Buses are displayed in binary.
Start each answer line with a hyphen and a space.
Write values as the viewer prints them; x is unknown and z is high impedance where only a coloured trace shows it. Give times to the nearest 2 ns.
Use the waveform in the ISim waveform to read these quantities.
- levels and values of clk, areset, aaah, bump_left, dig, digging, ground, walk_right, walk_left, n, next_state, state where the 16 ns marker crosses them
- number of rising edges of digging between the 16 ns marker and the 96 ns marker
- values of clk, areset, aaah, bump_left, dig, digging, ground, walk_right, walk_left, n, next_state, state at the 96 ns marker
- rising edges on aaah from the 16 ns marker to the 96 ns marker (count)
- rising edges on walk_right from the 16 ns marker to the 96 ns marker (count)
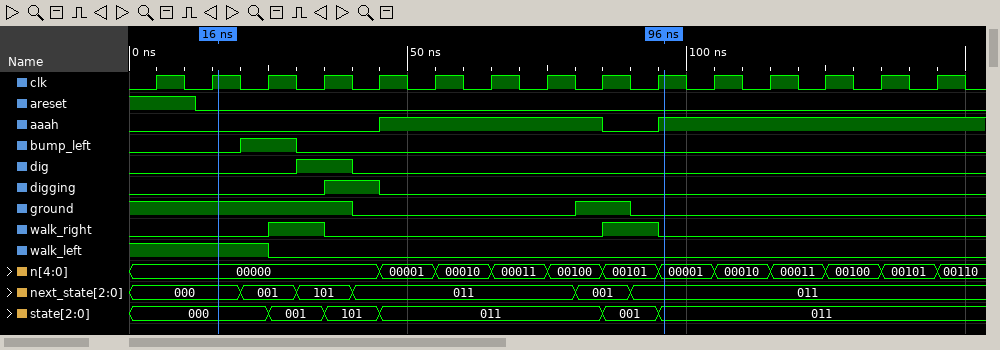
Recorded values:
- clk=1, areset=0, aaah=0, bump_left=0, dig=0, digging=0, ground=1, walk_right=0, walk_left=1, n=00000, next_state=000, state=000
- 1
- clk=1, areset=0, aaah=1, bump_left=0, dig=0, digging=0, ground=0, walk_right=0, walk_left=0, n=00001, next_state=011, state=011
- 2
- 2
